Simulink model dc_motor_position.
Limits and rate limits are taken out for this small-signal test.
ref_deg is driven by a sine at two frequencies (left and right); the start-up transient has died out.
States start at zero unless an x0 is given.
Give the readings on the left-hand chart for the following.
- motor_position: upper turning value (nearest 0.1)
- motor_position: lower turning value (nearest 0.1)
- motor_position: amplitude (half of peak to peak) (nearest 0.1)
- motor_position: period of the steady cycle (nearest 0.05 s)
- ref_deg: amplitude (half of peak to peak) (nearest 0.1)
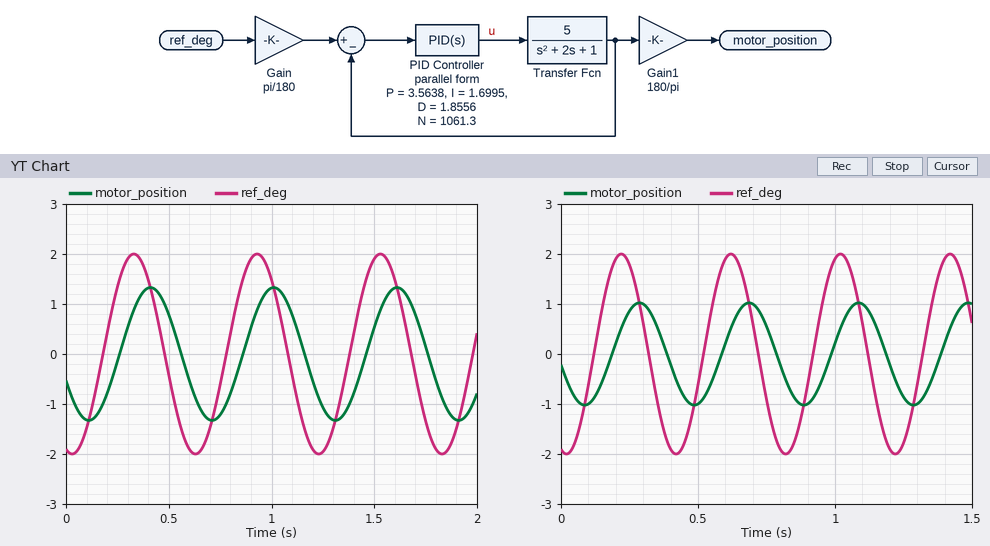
1.3
-1.3
1.3
0.60 s
2.0
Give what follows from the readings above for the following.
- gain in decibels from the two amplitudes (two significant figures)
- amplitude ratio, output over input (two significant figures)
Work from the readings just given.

-3.7 dB
0.65
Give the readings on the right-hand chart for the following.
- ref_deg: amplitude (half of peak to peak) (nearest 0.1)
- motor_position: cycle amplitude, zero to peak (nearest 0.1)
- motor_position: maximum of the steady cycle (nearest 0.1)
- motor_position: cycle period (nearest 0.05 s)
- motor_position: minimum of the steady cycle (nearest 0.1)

2.0
1.0
1.0
0.40 s
-1.0
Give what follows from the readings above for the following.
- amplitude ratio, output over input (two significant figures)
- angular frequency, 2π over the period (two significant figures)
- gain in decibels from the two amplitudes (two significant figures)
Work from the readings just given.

0.50
16 rad/s
-6.0 dB
